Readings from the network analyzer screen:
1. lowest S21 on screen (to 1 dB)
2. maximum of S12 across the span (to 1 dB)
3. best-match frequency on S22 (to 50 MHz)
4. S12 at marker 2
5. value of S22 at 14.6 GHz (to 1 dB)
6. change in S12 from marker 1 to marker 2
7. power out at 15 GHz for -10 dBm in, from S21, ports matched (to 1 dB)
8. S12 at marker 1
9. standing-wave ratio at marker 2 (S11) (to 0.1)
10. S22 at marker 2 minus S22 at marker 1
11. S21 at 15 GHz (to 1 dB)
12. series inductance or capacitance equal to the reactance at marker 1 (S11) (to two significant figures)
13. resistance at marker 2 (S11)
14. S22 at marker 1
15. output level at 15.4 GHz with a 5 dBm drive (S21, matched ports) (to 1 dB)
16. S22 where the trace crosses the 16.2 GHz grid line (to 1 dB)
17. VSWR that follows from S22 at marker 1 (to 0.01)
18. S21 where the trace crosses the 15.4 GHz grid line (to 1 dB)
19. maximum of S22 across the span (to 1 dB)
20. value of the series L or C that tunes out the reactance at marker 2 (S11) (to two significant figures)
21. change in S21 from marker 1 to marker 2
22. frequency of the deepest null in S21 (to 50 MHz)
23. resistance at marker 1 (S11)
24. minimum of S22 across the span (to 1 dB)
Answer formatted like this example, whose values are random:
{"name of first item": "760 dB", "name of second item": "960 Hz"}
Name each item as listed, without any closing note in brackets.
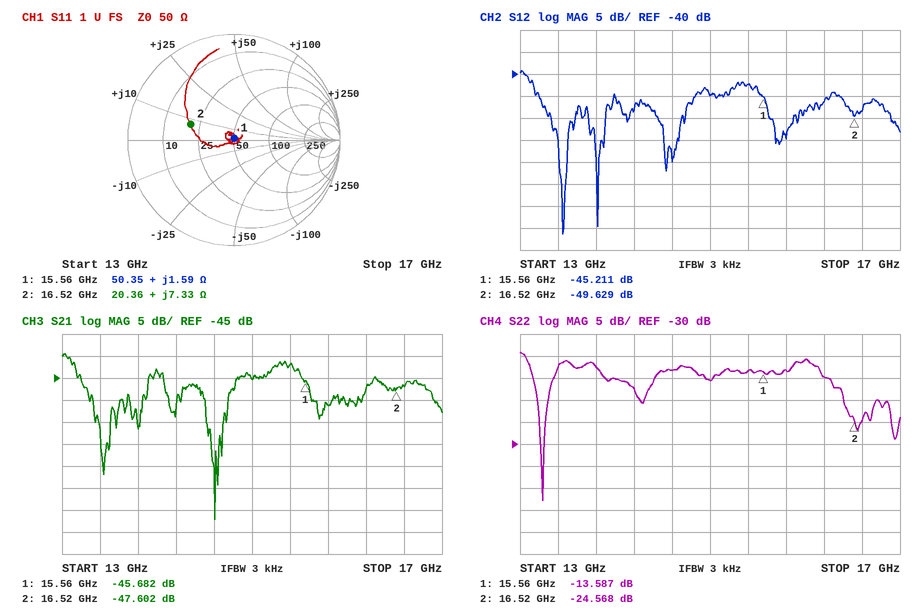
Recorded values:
{"lowest S21 on screen": "-77 dB", "maximum of S12 across the span": "-39 dB", "best-match frequency on S22": "13.25 GHz", "S12 at marker 2": "-49.629 dB", "value of S22 at 14.6 GHz": "-13 dB", "change in S12 from marker 1 to marker 2": "-4.418 dB", "power out at 15 GHz for -10 dBm in, from S21, ports matched": "-55 dBm", "S12 at marker 1": "-45.211 dB", "standing-wave ratio at marker 2 (S11)": "2.5", "S22 at marker 2 minus S22 at marker 1": "-10.981 dB", "S21 at 15 GHz": "-45 dB", "series inductance or capacitance equal to the reactance at marker 1 (S11)": "16 pH", "resistance at marker 2": "20.36 Ω", "S22 at marker 1": "-13.587 dB", "output level at 15.4 GHz with a 5 dBm drive (S21, matched ports)": "-37 dBm", "S22 where the trace crosses the 16.2 GHz grid line": "-15 dB", "VSWR that follows from S22 at marker 1": "1.53", "S21 where the trace crosses the 15.4 GHz grid line": "-42 dB", "maximum of S22 across the span": "-9 dB", "value of the series L or C that tunes out the reactance at marker 2 (S11)": "1.3 pF", "change in S21 from marker 1 to marker 2": "-1.920 dB", "frequency of the deepest null in S21": "14.60 GHz", "resistance at marker 1": "50.35 Ω", "minimum of S22 across the span": "-43 dB"}
